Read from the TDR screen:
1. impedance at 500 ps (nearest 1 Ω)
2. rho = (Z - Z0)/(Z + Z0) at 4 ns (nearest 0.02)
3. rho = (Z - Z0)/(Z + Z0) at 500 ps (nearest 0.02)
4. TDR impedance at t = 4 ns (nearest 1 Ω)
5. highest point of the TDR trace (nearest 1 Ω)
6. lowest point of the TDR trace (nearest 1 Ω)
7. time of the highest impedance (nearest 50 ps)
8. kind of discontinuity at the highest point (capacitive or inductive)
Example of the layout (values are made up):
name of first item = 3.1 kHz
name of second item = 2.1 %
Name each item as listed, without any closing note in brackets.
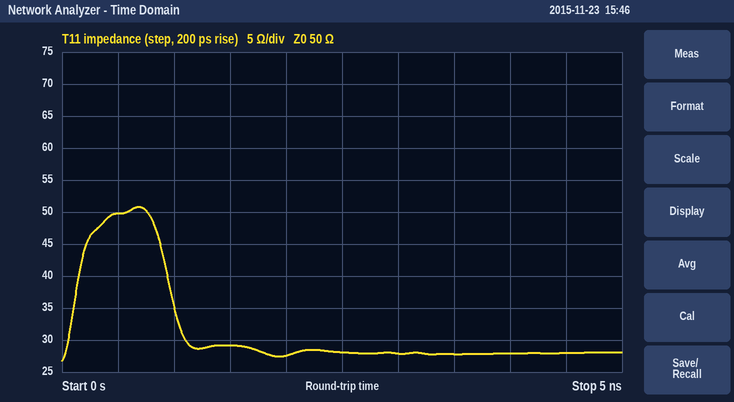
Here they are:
impedance at 500 ps = 50 Ω
rho = (Z - Z0)/(Z + Z0) at 4 ns = -0.28
rho = (Z - Z0)/(Z + Z0) at 500 ps = 0.00
TDR impedance at t = 4 ns = 28 Ω
highest point of the TDR trace = 51 Ω
lowest point of the TDR trace = 27 Ω
time of the highest impedance = 700 ps
kind of discontinuity at the highest point = inductive
